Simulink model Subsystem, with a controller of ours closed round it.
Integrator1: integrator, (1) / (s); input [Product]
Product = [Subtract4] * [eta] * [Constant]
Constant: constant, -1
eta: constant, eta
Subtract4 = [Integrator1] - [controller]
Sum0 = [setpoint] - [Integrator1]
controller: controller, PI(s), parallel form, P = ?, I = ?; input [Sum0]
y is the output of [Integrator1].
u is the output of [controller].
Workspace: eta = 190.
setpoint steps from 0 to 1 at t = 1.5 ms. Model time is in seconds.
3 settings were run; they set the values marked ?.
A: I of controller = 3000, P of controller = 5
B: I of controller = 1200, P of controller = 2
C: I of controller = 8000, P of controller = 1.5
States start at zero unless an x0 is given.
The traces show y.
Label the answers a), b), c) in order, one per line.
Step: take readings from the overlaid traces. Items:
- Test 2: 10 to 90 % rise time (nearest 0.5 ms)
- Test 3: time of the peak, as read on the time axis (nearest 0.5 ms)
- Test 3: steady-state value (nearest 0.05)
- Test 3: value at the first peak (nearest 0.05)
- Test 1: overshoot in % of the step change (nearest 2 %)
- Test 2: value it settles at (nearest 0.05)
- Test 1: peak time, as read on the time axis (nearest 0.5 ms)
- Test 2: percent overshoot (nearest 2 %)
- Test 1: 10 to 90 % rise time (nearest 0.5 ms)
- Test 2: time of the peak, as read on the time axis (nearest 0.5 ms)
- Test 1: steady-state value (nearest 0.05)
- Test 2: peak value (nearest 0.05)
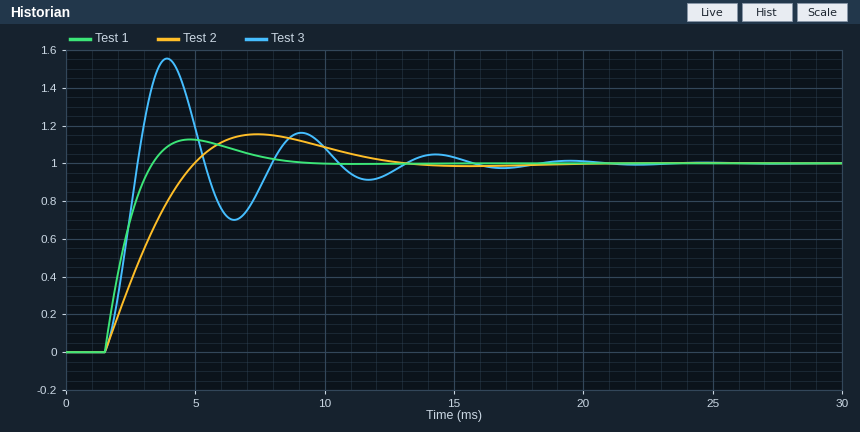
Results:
a) 2.5 ms
b) 4.0 ms
c) 1.00
d) 1.55
e) 12 %
f) 1.00
g) 5.0 ms
h) 16 %
i) 1.5 ms
j) 7.5 ms
k) 1.00
l) 1.15
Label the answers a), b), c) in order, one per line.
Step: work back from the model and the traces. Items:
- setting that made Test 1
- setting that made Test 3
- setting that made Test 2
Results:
a) A
b) C
c) B
